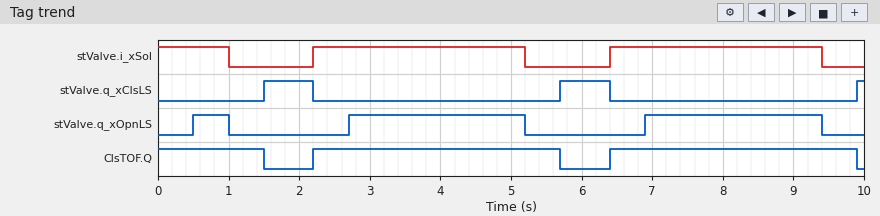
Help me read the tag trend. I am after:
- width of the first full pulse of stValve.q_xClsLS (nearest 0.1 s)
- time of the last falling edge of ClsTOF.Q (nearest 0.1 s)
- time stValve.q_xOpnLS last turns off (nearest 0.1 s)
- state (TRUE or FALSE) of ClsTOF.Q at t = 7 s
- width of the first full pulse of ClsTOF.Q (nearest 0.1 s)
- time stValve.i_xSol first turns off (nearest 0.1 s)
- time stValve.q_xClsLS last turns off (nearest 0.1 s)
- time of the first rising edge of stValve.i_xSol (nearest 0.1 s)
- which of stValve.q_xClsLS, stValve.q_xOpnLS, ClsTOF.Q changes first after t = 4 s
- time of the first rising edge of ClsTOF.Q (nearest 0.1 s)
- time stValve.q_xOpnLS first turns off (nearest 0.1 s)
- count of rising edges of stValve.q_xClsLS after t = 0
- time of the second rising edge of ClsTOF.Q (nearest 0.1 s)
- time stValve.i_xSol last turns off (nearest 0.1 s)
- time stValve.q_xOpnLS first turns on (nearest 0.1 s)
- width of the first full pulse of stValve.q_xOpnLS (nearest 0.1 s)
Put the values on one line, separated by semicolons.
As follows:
0.7 s; 9.9 s; 9.4 s; TRUE; 3.5 s; 1.0 s; 6.4 s; 2.2 s; stValve.q_xOpnLS; 2.2 s; 1.0 s; 3; 6.4 s; 9.4 s; 0.5 s; 0.5 s
